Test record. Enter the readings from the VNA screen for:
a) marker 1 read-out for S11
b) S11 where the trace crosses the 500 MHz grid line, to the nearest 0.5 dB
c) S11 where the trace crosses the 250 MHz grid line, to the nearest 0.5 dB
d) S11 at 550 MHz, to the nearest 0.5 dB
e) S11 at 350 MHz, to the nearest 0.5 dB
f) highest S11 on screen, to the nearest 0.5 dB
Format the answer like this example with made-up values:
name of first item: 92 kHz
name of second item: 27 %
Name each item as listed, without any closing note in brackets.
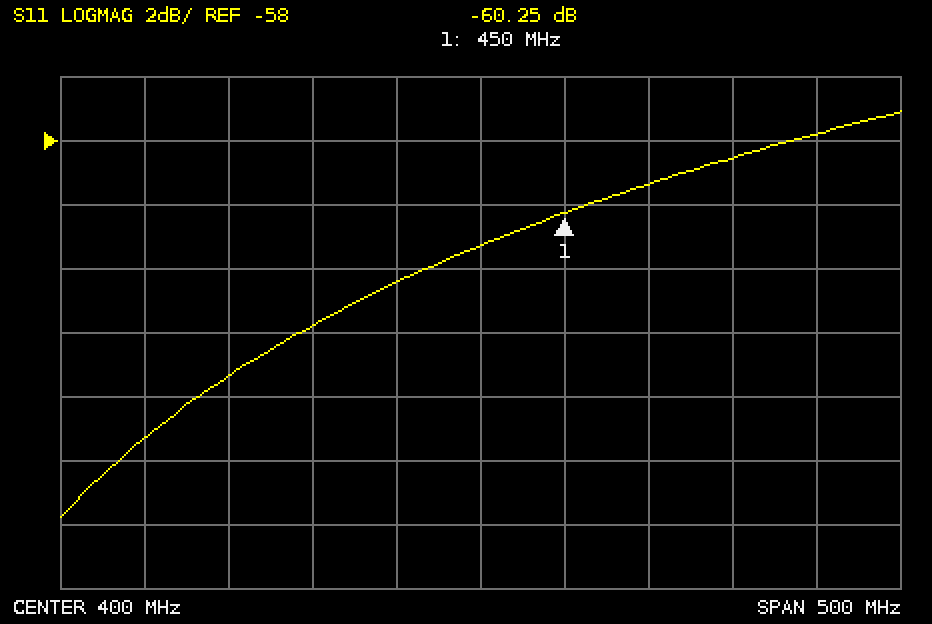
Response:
marker 1 read-out for S11: -60.25 dB
S11 where the trace crosses the 500 MHz grid line, to the nearest 0.5 dB: -59.5 dB
S11 where the trace crosses the 250 MHz grid line, to the nearest 0.5 dB: -65.5 dB
S11 at 550 MHz, to the nearest 0.5 dB: -58.5 dB
S11 at 350 MHz, to the nearest 0.5 dB: -62.5 dB
highest S11 on screen, to the nearest 0.5 dB: -57.0 dB
